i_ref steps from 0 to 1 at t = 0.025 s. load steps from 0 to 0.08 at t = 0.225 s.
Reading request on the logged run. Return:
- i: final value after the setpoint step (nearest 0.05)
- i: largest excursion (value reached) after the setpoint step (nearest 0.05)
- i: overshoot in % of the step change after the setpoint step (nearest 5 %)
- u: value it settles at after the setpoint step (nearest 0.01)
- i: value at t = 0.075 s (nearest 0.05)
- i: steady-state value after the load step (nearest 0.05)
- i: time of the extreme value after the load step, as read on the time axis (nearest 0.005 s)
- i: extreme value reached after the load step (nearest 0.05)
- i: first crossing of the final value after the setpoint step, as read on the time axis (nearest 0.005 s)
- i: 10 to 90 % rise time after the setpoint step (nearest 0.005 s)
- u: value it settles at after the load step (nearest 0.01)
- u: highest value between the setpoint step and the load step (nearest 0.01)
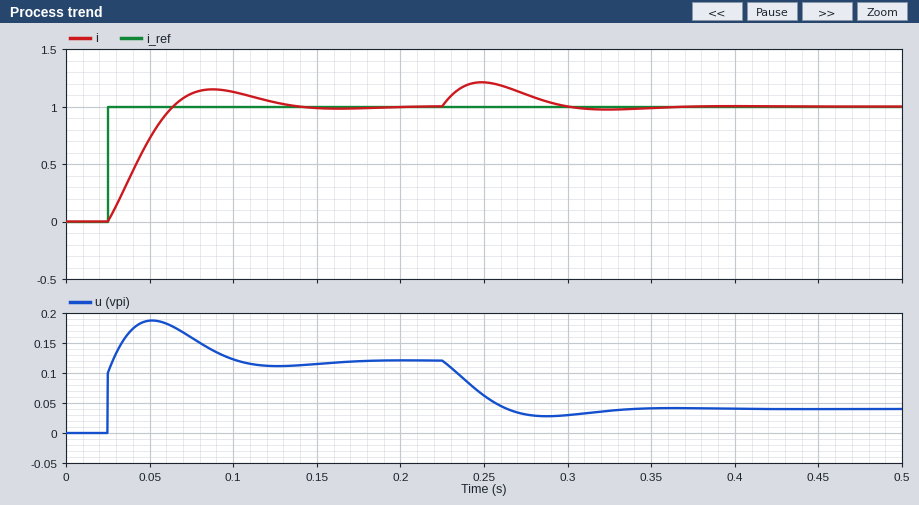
1.00
1.15
15 %
0.12
1.10
1.00
0.250 s
1.20
0.065 s
0.030 s
0.04
0.19
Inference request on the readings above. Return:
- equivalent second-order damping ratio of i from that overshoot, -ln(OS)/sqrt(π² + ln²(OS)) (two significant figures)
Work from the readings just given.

0.52
